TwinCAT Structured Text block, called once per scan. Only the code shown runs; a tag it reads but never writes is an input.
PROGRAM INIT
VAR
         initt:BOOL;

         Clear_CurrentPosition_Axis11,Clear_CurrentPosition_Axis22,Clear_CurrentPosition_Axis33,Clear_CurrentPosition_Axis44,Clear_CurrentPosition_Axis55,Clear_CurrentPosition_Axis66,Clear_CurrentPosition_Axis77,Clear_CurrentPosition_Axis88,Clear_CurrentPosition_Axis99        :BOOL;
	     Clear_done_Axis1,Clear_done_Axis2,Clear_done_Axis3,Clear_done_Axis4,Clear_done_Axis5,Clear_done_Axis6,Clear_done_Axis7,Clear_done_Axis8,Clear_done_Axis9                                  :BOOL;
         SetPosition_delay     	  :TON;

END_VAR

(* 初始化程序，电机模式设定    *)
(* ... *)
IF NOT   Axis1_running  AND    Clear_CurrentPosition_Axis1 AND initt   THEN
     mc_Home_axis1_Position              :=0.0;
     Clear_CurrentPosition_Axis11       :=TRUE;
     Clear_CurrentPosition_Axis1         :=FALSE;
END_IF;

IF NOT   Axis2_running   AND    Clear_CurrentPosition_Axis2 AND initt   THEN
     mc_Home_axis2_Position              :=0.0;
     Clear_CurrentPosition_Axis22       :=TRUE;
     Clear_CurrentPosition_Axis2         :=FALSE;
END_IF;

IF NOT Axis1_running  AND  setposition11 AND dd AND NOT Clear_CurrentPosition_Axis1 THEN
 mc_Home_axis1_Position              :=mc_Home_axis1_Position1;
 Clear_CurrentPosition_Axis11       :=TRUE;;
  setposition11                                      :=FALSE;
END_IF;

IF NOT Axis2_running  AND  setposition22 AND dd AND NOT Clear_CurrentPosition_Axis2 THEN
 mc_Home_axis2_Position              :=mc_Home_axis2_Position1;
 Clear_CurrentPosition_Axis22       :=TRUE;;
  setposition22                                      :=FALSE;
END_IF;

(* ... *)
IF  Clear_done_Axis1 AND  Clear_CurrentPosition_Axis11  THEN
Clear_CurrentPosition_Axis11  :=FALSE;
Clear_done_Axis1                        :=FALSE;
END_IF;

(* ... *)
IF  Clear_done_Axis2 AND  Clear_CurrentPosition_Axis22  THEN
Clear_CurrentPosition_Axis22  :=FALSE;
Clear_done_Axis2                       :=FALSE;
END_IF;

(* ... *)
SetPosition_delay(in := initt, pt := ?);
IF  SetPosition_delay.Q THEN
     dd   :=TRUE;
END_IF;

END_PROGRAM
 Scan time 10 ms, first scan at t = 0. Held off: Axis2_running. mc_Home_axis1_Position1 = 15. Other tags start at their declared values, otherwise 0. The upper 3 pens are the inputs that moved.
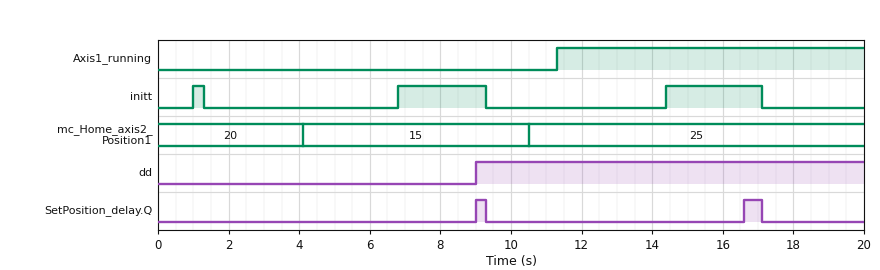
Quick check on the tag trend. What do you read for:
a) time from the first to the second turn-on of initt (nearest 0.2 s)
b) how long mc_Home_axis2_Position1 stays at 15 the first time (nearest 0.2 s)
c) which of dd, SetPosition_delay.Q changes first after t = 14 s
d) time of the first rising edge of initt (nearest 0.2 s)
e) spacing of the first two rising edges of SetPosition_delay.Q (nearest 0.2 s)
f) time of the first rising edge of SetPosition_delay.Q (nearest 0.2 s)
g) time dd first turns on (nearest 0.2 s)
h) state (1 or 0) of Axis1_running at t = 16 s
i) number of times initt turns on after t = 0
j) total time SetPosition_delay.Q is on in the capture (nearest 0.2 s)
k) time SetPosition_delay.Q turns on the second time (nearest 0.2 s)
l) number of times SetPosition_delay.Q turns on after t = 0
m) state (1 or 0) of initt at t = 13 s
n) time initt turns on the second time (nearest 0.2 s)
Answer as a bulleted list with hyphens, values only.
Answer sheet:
- 5.8 s
- 6.4 s
- SetPosition_delay.Q
- 1.0 s
- 7.6 s
- 9.0 s
- 9.0 s
- 1
- 3
- 0.8 s
- 16.6 s
- 2
- 0
- 6.8 s
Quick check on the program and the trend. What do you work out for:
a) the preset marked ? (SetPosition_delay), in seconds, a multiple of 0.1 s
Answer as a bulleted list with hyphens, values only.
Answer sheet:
- 2.2 s
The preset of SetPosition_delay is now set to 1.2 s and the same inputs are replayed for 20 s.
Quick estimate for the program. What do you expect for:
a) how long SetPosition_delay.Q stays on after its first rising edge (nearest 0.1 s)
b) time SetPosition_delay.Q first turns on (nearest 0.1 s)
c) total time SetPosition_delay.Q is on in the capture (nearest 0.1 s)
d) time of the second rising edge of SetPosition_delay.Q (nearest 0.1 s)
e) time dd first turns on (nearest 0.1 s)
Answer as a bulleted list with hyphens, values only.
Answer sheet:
- 1.3 s
- 8.0 s
- 2.8 s
- 15.6 s
- 8.0 s
